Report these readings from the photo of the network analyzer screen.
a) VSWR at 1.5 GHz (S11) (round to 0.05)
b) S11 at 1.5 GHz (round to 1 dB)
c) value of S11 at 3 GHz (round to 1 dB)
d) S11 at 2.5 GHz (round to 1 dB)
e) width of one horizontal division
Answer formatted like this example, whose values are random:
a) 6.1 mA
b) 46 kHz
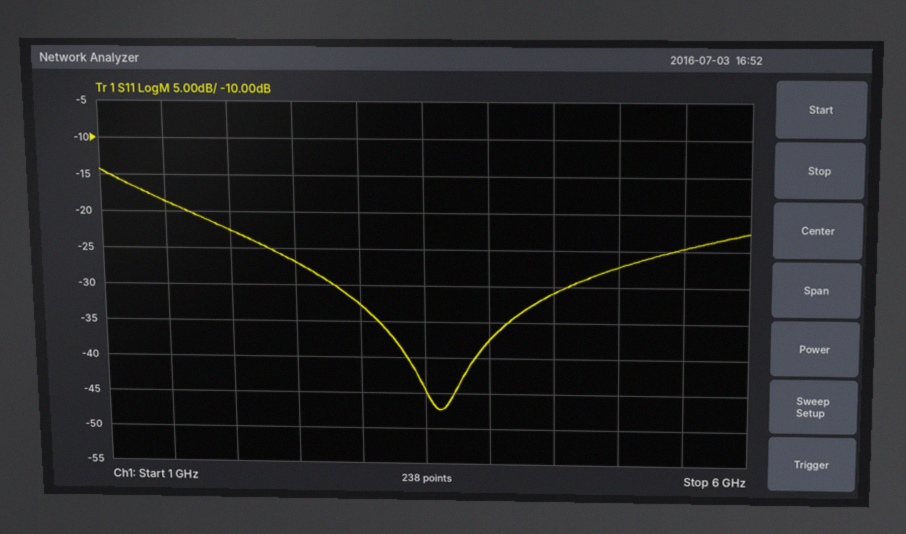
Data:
a) 1.25
b) -19 dB
c) -33 dB
d) -27 dB
e) 500 MHz
